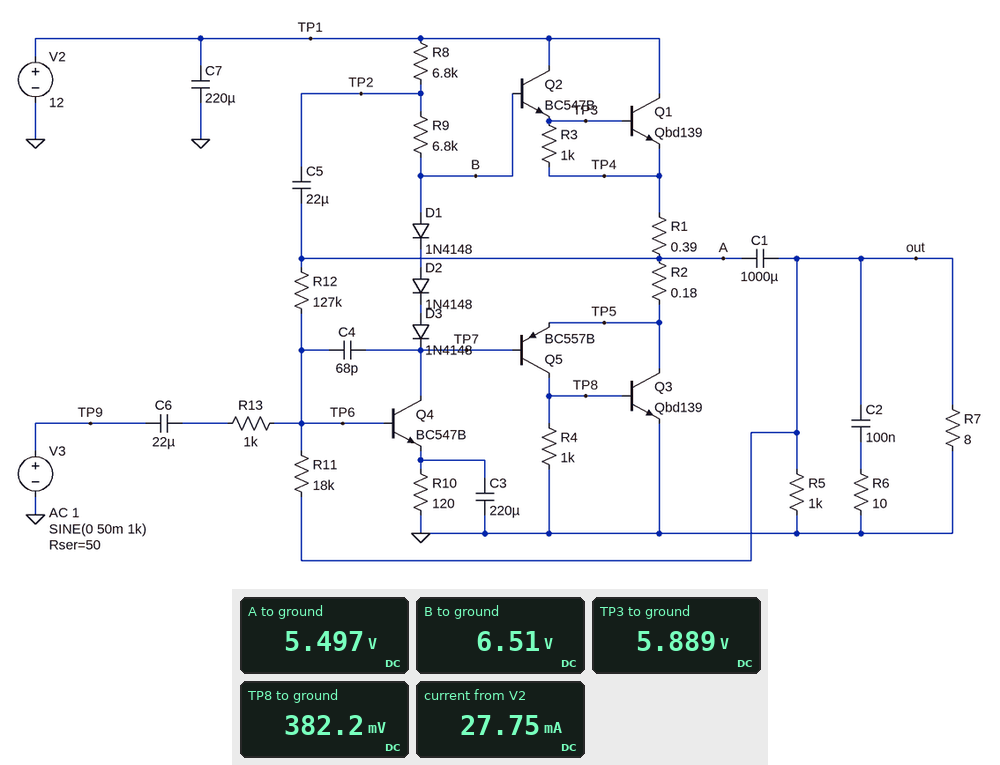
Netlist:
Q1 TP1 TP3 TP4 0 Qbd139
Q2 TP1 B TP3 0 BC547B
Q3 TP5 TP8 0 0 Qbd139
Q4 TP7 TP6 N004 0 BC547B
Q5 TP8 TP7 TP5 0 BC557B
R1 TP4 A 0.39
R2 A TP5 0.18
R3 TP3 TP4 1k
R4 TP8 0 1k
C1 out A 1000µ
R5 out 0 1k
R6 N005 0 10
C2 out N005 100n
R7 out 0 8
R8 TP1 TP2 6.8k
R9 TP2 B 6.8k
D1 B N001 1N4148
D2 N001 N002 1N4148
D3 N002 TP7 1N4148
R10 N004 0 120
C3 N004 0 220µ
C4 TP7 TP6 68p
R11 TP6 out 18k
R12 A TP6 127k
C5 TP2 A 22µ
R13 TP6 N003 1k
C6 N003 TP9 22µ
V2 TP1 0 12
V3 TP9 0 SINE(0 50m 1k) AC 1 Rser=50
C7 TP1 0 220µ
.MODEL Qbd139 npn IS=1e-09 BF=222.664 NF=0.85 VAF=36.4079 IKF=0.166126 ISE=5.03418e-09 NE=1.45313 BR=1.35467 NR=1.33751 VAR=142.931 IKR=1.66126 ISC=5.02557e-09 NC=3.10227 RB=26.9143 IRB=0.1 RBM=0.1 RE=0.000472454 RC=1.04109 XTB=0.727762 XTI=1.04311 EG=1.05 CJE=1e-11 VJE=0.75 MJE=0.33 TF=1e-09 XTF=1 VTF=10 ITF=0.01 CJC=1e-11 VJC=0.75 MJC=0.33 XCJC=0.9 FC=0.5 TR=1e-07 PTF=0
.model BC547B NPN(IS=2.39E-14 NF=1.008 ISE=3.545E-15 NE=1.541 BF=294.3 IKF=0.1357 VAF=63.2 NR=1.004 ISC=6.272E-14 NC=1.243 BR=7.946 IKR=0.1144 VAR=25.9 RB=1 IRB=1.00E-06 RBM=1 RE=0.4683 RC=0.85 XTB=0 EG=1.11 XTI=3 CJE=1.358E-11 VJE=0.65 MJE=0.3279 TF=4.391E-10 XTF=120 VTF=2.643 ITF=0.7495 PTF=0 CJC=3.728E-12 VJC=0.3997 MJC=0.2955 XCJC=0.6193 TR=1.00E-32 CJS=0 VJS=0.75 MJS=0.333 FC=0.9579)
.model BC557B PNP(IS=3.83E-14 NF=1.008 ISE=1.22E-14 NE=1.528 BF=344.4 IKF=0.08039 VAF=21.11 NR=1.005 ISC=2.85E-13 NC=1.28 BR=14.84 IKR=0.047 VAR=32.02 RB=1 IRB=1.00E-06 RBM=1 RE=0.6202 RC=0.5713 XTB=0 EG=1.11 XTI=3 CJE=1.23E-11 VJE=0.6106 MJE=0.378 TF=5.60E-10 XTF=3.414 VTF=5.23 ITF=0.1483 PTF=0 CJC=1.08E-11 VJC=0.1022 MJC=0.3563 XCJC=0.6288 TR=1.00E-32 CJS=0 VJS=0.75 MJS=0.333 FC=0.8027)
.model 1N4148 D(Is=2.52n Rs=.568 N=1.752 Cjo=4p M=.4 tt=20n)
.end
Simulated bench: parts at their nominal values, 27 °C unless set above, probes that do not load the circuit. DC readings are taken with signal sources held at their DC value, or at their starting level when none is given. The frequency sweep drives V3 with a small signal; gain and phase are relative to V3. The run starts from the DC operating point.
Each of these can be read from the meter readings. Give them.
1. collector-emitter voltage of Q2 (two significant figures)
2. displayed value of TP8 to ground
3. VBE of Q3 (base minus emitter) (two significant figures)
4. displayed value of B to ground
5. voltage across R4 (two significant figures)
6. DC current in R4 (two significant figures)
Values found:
6.1 V
382.2 mV
380 mV
6.51 V
380 mV
380 µA
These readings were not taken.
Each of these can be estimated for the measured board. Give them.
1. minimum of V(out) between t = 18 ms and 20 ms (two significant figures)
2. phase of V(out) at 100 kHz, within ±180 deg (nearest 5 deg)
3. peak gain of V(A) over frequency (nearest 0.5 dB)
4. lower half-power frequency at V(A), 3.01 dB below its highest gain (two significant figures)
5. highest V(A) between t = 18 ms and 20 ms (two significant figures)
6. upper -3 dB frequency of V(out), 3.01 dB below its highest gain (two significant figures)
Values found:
-730 mV
140 deg
30.0 dB
2.2 Hz
6.2 V
130 kHz
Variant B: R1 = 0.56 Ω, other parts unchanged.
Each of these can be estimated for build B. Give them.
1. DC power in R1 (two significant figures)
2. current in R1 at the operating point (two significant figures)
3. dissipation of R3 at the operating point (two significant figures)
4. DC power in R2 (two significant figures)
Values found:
370 µW
26 mA
140 µW
120 µW
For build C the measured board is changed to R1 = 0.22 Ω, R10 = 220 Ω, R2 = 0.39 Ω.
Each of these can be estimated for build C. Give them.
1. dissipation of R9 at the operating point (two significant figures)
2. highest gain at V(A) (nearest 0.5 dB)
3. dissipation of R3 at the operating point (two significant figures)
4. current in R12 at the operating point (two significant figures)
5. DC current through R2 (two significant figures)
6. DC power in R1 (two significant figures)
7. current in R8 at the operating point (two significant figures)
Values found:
1.0 mW
30.5 dB
140 µW
40 µA
24 mA
130 µW
380 µA
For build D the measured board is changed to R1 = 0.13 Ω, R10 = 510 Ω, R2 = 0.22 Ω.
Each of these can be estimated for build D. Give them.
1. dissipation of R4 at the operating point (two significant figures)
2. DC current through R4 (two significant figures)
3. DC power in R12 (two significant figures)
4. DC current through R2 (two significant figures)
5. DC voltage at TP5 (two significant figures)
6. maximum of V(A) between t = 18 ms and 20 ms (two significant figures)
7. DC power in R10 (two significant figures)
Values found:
140 µW
370 µA
250 µW
20 mA
6.4 V
7.1 V
58 µW
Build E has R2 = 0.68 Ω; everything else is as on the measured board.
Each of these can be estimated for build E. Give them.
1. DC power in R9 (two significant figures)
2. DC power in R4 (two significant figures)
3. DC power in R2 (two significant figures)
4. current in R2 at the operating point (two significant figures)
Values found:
1.1 mW
140 µW
360 µW
23 mA
